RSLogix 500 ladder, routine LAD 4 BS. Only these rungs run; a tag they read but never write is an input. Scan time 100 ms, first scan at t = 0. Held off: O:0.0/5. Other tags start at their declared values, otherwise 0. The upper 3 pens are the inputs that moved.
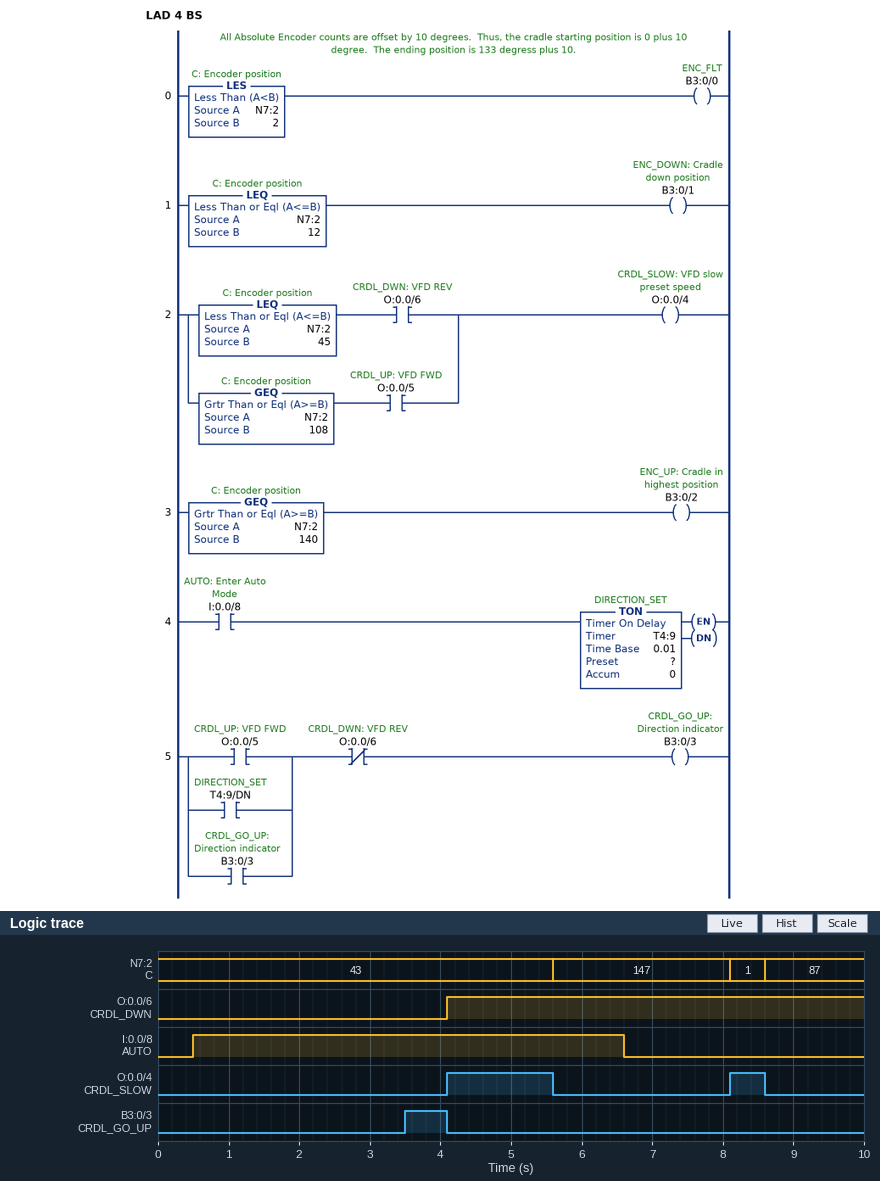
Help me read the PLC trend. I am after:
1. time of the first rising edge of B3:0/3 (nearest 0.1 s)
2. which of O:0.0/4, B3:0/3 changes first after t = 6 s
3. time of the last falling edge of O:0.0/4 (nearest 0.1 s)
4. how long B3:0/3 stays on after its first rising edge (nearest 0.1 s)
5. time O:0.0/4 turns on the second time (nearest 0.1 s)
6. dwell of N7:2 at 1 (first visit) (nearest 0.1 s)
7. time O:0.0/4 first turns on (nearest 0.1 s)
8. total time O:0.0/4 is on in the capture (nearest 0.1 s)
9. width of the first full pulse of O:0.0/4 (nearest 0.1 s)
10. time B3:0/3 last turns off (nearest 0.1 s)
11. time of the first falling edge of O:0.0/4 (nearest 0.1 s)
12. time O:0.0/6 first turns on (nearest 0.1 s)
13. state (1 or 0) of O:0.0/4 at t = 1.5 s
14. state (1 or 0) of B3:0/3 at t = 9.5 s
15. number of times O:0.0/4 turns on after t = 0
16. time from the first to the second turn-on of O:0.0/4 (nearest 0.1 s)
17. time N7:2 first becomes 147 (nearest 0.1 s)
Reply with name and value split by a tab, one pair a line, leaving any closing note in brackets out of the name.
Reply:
time of the first rising edge of B3:0/3	3.5 s
which of O:0.0/4, B3:0/3 changes first after t = 6 s	O:0.0/4
time of the last falling edge of O:0.0/4	8.6 s
how long B3:0/3 stays on after its first rising edge	0.6 s
time O:0.0/4 turns on the second time	8.1 s
dwell of N7:2 at 1 (first visit)	0.5 s
time O:0.0/4 first turns on	4.1 s
total time O:0.0/4 is on in the capture	2.0 s
width of the first full pulse of O:0.0/4	1.5 s
time B3:0/3 last turns off	4.1 s
time of the first falling edge of O:0.0/4	5.6 s
time O:0.0/6 first turns on	4.1 s
state (1 or 0) of O:0.0/4 at t = 1.5 s	0
state (1 or 0) of B3:0/3 at t = 9.5 s	0
number of times O:0.0/4 turns on after t = 0	2
time from the first to the second turn-on of O:0.0/4	4.0 s
time N7:2 first becomes 147	5.6 s
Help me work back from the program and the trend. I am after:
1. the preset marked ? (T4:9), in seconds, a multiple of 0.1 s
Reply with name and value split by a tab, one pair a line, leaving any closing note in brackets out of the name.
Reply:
the preset marked ? (T4:9), in seconds, a multiple of 0.1 s	3.0 s
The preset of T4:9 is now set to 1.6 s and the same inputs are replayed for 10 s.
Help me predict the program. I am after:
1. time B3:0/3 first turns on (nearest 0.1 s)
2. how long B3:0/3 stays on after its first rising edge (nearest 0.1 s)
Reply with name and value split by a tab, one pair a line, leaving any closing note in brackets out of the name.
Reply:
time B3:0/3 first turns on	2.1 s
how long B3:0/3 stays on after its first rising edge	2.0 s
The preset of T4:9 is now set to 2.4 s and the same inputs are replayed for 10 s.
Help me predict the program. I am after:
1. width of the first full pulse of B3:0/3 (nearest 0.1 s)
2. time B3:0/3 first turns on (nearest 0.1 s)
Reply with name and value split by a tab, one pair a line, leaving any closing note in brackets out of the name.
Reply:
width of the first full pulse of B3:0/3	1.2 s
time B3:0/3 first turns on	2.9 s
